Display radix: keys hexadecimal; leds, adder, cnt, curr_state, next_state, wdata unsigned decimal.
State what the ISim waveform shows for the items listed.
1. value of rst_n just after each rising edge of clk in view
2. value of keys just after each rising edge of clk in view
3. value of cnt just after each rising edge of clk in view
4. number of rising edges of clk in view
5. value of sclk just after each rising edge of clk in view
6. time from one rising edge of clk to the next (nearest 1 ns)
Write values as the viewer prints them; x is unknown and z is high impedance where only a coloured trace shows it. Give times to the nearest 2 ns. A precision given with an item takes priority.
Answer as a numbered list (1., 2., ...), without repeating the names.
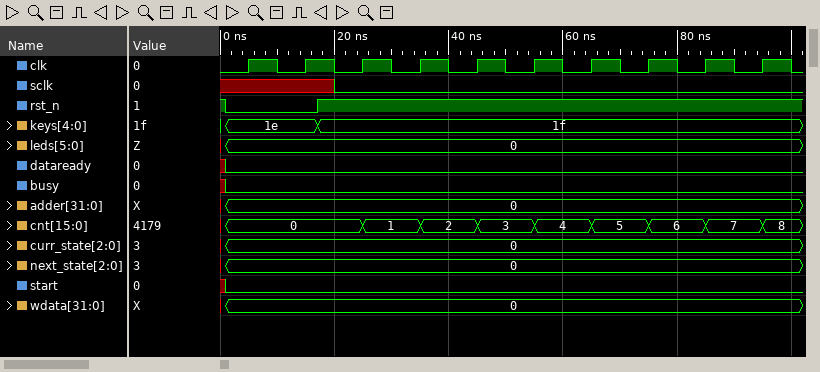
1. 0 0 1 1 1 1 1 1 1 1
2. 1e, 1e, 1f, 1f, 1f, 1f, 1f, 1f, 1f, 1f
3. 0, 0, 1, 2, 3, 4, 5, 6, 7, 8
4. 10
5. x x 0 0 0 0 0 0 0 0
6. 10 ns
